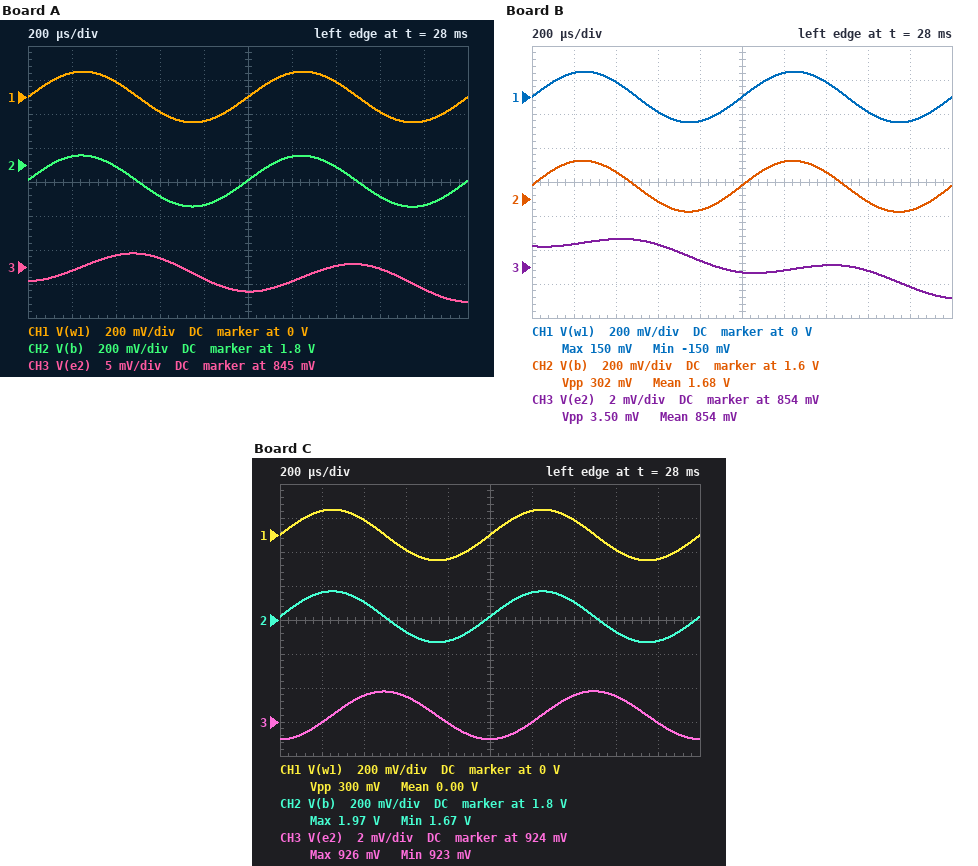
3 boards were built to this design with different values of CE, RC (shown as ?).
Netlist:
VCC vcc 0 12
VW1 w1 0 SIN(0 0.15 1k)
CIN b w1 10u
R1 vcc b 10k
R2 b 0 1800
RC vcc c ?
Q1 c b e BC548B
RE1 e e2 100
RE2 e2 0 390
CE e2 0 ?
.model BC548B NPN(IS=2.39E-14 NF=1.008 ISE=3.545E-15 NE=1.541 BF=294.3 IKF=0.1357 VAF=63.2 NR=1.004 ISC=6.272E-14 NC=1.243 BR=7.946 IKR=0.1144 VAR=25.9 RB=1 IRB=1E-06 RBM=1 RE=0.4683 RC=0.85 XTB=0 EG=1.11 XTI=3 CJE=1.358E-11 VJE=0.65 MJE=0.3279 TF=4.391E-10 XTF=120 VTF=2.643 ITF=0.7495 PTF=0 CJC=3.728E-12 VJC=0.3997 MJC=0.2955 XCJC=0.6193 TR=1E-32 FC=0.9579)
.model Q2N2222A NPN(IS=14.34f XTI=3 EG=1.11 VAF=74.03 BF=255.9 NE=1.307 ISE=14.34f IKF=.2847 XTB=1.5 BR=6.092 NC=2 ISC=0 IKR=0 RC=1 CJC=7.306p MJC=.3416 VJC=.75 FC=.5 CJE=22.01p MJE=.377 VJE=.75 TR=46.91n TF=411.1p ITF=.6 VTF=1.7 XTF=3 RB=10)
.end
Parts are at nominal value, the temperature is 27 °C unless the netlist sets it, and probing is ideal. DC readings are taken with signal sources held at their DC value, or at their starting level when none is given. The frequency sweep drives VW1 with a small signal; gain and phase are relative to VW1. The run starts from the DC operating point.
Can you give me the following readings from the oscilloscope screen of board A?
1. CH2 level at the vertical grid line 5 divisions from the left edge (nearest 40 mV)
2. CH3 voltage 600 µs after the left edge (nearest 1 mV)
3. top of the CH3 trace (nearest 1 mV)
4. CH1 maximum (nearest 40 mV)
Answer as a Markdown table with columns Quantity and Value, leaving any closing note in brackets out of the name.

| Quantity | Value |
|---|---|
| CH2 level at the vertical grid line 5 divisions from the left edge | 1.72 V |
| CH3 voltage 600 µs after the left edge | 846 mV |
| top of the CH3 trace | 847 mV |
| CH1 maximum | 160 mV |
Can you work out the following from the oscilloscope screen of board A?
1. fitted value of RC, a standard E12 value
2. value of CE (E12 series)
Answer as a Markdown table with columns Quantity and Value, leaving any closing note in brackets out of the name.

| Quantity | Value |
|---|---|
| fitted value of RC, a standard E12 value | 3.9 kΩ |
| value of CE | 82 µF |
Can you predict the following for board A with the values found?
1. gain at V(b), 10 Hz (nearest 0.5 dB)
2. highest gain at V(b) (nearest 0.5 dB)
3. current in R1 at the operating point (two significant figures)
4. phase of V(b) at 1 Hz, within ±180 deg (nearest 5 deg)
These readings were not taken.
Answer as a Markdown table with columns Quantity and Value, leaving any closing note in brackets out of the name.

| Quantity | Value |
|---|---|
| gain at V(b), 10 Hz | -3.5 dB |
| highest gain at V(b) | 0 dB |
| current in R1 at the operating point | 1.0 mA |
| phase of V(b) at 1 Hz, within ±180 deg | 85 deg |
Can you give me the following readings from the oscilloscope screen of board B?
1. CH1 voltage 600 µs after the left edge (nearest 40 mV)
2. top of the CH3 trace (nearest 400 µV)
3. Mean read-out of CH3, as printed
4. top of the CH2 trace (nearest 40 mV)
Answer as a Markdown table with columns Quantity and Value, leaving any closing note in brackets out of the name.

| Quantity | Value |
|---|---|
| CH1 voltage 600 µs after the left edge | -80 mV |
| top of the CH3 trace | 855.6 mV |
| Mean read-out of CH3, as printed | 854 mV |
| top of the CH2 trace | 1.84 V |
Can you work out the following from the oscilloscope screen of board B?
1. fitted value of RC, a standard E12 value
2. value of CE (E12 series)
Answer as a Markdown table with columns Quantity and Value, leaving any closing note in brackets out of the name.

| Quantity | Value |
|---|---|
| fitted value of RC, a standard E12 value | 4.7 kΩ |
| value of CE | 330 µF |
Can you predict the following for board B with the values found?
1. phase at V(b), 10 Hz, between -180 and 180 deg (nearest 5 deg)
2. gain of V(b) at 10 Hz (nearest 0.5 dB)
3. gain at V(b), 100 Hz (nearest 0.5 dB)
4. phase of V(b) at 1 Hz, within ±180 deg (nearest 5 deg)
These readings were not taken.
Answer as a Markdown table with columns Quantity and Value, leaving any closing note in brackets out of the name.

| Quantity | Value |
|---|---|
| phase at V(b), 10 Hz, between -180 and 180 deg | 70 deg |
| gain of V(b) at 10 Hz | -18.0 dB |
| gain at V(b), 100 Hz | -2.5 dB |
| phase of V(b) at 1 Hz, within ±180 deg | 70 deg |
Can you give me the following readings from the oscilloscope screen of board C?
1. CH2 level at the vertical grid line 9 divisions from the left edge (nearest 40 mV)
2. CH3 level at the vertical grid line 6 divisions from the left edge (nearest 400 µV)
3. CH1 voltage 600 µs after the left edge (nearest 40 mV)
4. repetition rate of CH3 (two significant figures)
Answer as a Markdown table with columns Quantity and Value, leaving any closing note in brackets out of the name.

| Quantity | Value |
|---|---|
| CH2 level at the vertical grid line 9 divisions from the left edge | 1.68 V |
| CH3 level at the vertical grid line 6 divisions from the left edge | 924.0 mV |
| CH1 voltage 600 µs after the left edge | -80 mV |
| repetition rate of CH3 | 1.0 kHz |
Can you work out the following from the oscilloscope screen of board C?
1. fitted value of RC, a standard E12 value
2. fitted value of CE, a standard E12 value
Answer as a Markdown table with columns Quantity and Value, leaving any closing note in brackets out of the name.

| Quantity | Value |
|---|---|
| fitted value of RC, a standard E12 value | 1.2 kΩ |
| fitted value of CE, a standard E12 value | 150 µF |
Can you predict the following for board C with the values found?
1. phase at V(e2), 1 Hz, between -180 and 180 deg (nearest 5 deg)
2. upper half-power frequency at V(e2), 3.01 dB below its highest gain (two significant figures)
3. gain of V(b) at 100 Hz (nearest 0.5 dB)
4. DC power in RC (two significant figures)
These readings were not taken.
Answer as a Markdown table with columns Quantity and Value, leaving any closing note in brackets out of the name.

| Quantity | Value |
|---|---|
| phase at V(e2), 1 Hz, between -180 and 180 deg | 80 deg |
| upper half-power frequency at V(e2), 3.01 dB below its highest gain | 28 Hz |
| gain of V(b) at 100 Hz | 0 dB |
| DC power in RC | 6.7 mW |
